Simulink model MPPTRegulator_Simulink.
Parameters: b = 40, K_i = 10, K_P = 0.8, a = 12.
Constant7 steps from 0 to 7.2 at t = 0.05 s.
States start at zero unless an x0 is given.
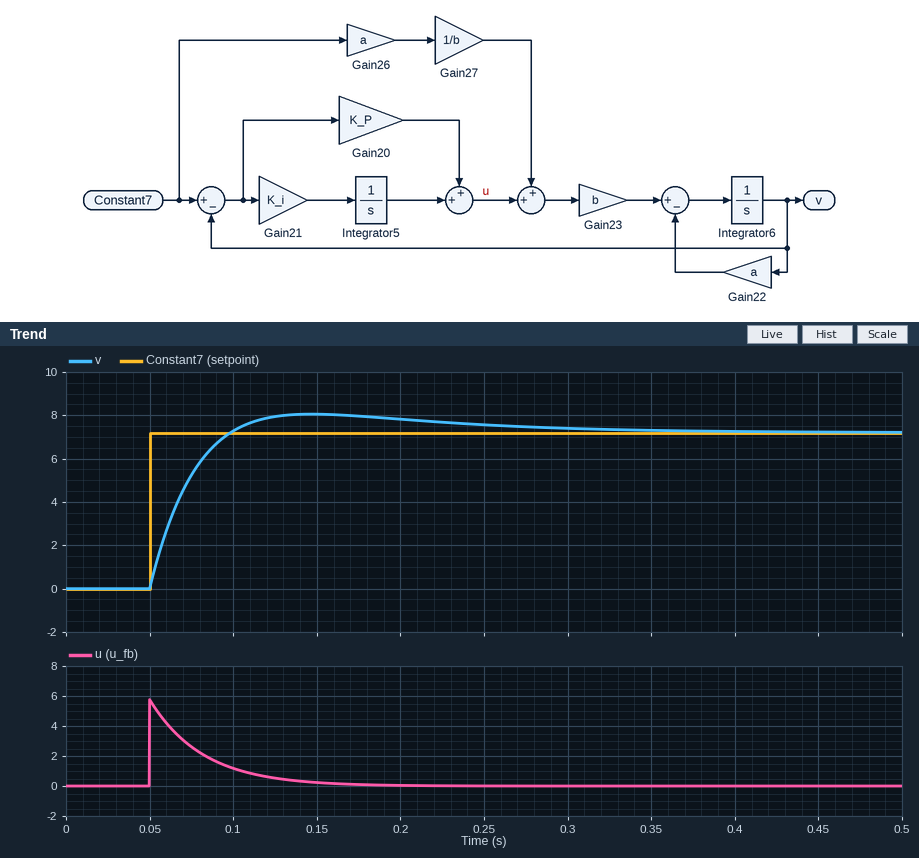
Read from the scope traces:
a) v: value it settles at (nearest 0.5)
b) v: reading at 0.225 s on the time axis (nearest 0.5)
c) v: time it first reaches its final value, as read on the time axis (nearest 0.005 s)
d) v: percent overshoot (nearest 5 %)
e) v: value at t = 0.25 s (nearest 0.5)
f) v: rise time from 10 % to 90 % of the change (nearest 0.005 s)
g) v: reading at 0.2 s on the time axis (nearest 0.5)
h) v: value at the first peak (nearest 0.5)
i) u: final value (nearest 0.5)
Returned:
7.0
7.5
0.100 s
10 %
7.5
0.035 s
8.0
8.0
0.0
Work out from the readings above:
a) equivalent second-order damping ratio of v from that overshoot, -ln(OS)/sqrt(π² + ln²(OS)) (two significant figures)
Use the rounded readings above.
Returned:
0.59
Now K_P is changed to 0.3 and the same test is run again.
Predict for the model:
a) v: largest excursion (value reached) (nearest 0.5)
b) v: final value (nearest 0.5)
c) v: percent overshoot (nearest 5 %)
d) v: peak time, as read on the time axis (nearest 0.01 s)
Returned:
9.0
7.0
25 %
0.17 s
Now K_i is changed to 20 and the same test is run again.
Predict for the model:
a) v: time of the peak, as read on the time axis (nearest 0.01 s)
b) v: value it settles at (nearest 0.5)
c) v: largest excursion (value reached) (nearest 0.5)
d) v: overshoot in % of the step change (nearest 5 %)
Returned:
0.13 s
7.0
8.5
20 %
